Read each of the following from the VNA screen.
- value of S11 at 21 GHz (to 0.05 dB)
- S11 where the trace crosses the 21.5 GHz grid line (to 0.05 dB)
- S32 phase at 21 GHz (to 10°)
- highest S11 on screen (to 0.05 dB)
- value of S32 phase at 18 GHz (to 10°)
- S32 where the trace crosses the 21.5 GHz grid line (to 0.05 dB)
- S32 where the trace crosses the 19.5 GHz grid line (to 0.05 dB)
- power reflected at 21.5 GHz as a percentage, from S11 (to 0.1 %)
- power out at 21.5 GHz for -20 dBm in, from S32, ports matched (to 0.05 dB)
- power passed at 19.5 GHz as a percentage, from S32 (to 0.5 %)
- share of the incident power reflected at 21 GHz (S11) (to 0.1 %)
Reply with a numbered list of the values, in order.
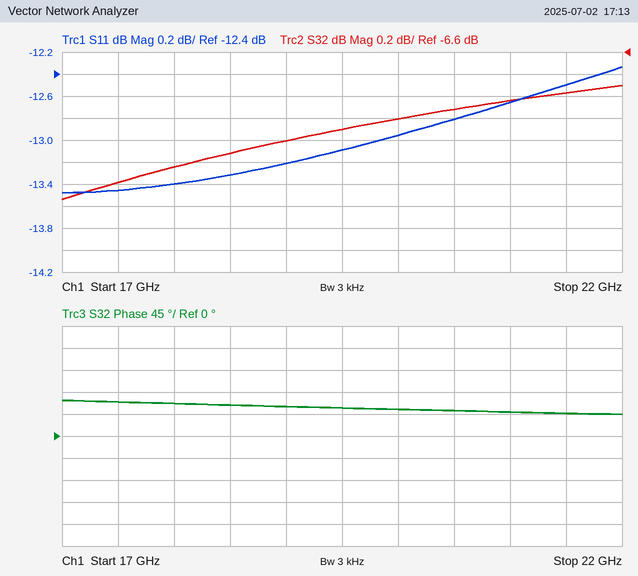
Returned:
1. -12.65 dB
2. -12.50 dB
3. 50°
4. -12.35 dB
5. 70°
6. -6.95 dB
7. -7.30 dB
8. 5.6 %
9. -26.95 dBm
10. 18.5 %
11. 5.4 %
